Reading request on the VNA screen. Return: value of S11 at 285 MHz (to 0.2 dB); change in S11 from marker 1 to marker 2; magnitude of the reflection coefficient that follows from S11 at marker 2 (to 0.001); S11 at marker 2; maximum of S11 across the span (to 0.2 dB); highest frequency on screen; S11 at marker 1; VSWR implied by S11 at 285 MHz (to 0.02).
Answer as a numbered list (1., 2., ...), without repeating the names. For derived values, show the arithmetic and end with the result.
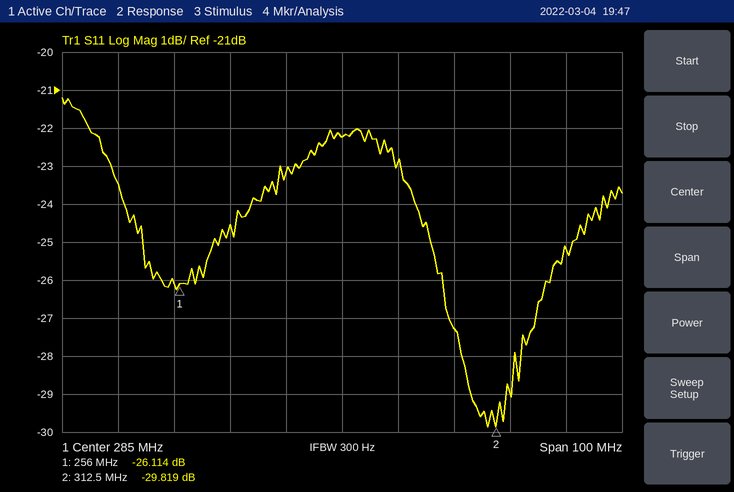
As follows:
1. -22.2 dB
2. -29.819 − (-26.114) = -3.705 dB
3. 10^(-29.819/20) ≈ 0.032
4. -29.819 dB
5. -21.2 dB
6. 335 MHz
7. -26.114 dB
8. |Γ| = 10^(-22.2/20) = 0.0776; VSWR = (1 + 0.0776)/(1 − 0.0776) ≈ 1.17, so 1.16 to the nearest 0.02
